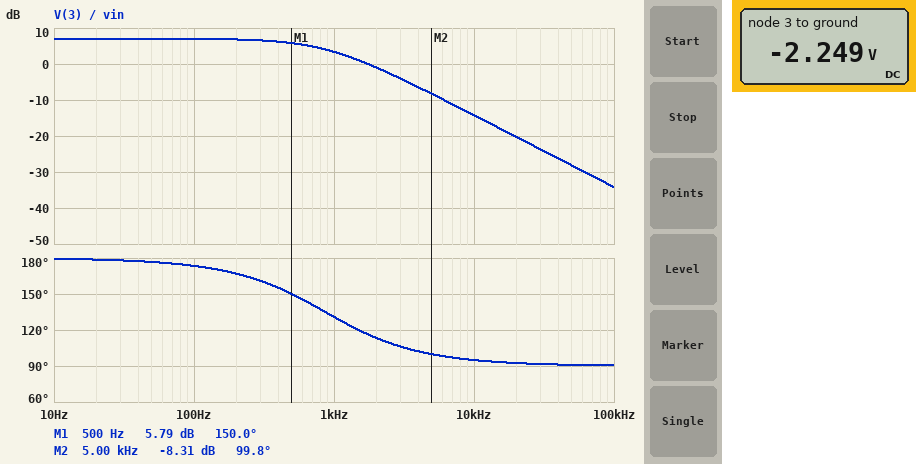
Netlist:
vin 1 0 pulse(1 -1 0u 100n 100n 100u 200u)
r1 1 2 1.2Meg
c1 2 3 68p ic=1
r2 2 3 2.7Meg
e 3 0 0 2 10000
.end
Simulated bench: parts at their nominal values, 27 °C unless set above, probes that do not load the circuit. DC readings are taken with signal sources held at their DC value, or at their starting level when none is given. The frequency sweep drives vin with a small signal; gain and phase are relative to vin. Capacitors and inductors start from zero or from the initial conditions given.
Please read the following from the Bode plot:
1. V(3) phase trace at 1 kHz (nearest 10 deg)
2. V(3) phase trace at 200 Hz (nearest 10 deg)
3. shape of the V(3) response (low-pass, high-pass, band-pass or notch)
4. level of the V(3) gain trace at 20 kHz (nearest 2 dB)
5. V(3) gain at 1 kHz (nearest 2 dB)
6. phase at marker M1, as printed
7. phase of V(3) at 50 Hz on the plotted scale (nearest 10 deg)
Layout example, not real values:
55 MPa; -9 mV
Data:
130 deg; 170 deg; low-pass; -20 dB; 4 dB; 150.0 deg; 180 deg
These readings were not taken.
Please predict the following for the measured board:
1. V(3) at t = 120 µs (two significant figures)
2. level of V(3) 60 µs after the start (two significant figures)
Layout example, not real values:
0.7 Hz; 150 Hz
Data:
98 mV; -95 mV
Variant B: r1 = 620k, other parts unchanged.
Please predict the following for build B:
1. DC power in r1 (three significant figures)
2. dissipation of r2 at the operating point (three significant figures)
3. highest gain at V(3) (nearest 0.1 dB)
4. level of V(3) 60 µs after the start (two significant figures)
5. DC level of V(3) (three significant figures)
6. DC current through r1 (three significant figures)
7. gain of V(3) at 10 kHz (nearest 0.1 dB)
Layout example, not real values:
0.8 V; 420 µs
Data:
1.61 µW; 7.02 µW; 12.8 dB; 490 mV; -4.35 V; 1.61 µA; -8.5 dB
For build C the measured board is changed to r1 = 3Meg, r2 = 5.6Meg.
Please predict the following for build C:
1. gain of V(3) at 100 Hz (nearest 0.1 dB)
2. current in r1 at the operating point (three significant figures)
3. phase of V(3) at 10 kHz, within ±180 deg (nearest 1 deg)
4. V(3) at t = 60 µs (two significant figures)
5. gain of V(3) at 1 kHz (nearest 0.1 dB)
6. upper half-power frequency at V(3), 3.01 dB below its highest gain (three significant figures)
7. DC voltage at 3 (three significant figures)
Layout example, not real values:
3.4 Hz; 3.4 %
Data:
5.2 dB; 333 nA; 92 deg; -580 mV; -2.9 dB; 418 Hz; -1.87 V
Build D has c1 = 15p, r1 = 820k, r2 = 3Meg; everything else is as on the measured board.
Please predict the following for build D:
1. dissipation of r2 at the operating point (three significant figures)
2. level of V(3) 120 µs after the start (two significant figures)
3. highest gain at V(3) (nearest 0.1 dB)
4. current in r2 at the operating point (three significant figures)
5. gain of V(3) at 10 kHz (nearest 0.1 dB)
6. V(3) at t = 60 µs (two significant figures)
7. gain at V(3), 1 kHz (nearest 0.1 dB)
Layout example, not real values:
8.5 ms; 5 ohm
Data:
4.46 µW; 720 mV; 11.3 dB; 1.22 µA; 1.7 dB; 2.4 V; 10.9 dB
